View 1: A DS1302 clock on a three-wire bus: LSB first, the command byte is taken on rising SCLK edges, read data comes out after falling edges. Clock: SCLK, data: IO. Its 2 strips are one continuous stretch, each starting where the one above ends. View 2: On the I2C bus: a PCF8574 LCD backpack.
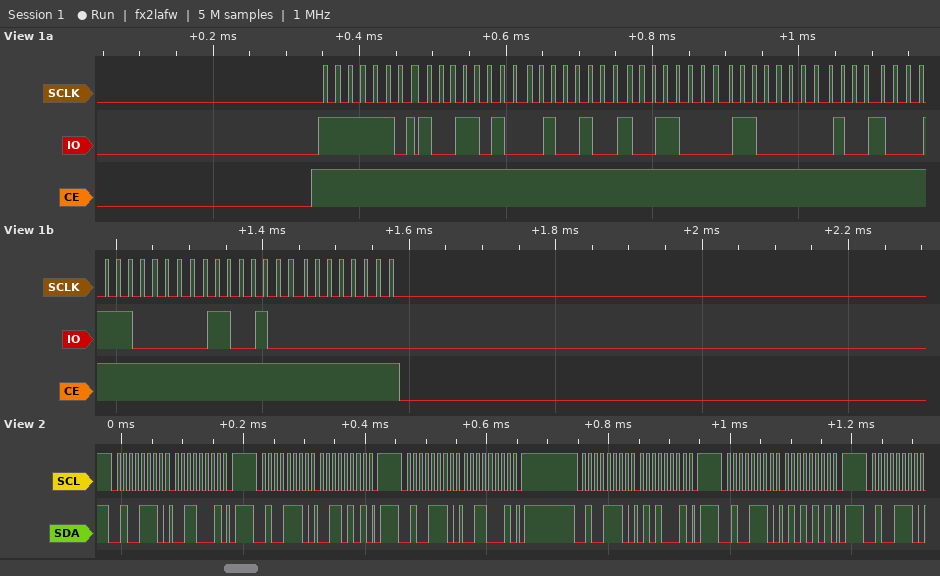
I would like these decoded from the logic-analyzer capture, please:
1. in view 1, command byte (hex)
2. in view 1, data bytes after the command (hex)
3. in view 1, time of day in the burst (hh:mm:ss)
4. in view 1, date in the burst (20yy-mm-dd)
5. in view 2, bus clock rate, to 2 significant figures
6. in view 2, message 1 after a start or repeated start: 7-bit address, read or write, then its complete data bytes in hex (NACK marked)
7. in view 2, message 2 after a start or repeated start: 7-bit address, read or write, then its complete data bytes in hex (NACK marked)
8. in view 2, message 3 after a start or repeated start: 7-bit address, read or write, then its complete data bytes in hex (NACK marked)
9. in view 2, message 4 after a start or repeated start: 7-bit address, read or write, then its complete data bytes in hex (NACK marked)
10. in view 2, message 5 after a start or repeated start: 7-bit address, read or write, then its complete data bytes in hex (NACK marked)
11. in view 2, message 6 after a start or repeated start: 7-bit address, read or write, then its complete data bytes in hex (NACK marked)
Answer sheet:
0xBF
59 24 19 06 12 07 26 00
19:24:59
2026-12-06
100 kHz
0x27 write: 31
0x27 write: 35
0x27 write: 31
0x27 write: 51
0x27 write: 55
0x27 write
